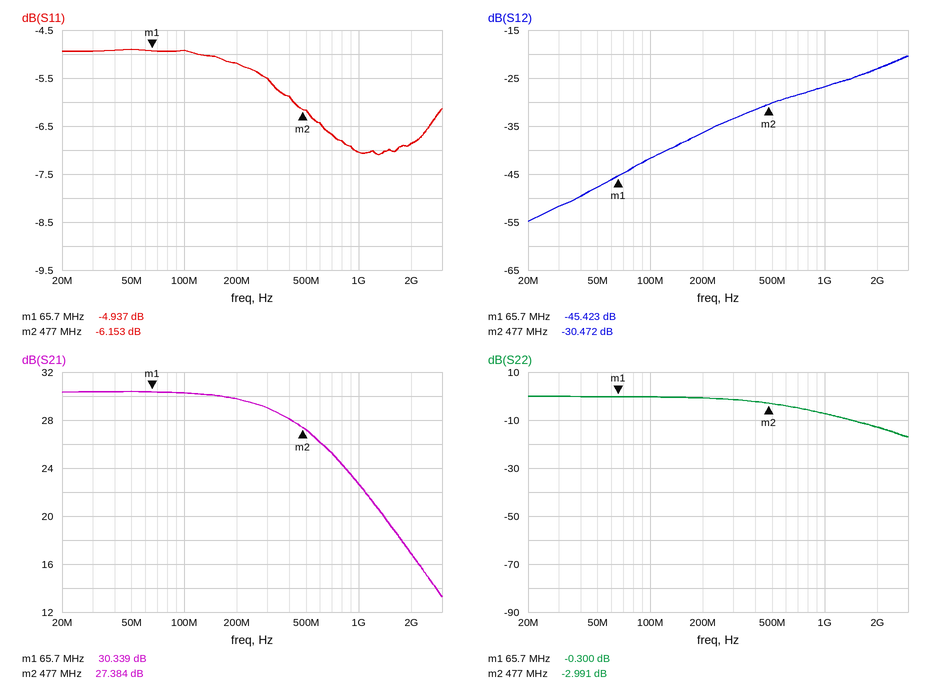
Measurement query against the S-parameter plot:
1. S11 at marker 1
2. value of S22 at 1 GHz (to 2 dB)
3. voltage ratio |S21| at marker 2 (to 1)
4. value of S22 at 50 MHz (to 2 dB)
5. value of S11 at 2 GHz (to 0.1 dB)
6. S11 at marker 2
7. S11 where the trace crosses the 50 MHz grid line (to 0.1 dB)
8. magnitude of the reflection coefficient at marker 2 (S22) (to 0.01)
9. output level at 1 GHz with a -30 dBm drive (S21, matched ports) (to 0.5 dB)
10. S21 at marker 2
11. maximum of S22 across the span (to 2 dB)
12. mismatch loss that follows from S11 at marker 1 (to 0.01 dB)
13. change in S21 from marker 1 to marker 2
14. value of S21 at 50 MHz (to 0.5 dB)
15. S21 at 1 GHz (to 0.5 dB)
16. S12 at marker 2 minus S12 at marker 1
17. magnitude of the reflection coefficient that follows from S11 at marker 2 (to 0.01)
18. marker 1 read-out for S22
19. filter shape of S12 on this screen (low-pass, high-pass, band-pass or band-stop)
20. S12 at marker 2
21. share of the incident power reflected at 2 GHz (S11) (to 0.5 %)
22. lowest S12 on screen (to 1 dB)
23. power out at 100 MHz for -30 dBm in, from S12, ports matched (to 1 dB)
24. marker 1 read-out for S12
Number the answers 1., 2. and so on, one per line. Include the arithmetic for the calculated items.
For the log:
1. -4.937 dB
2. -8 dB
3. 10^(27.384/20) ≈ 23
4. 0 dB
5. -6.9 dB
6. -6.153 dB
7. -4.9 dB
8. 10^(-2.991/20) ≈ 0.71
9. -30 dBm + (22.5 dB) = -7.5 dBm
10. 27.384 dB
11. 0 dB
12. −10 log10(1 − 10^(-4.937/10)) ≈ 1.68 dB
13. 27.384 − (30.339) = -2.955 dB
14. 30.5 dB
15. 22.5 dB
16. -30.472 − (-45.423) = 14.951 dB
17. 10^(-6.153/20) ≈ 0.49
18. -0.300 dB
19. high-pass
20. -30.472 dB
21. 10^(-6.9/10) ≈ 20.4 %, so 20.5 % to the nearest 0.5 %
22. -55 dB
23. -30 dBm + (-42 dB) = -72 dBm
24. -45.423 dB
